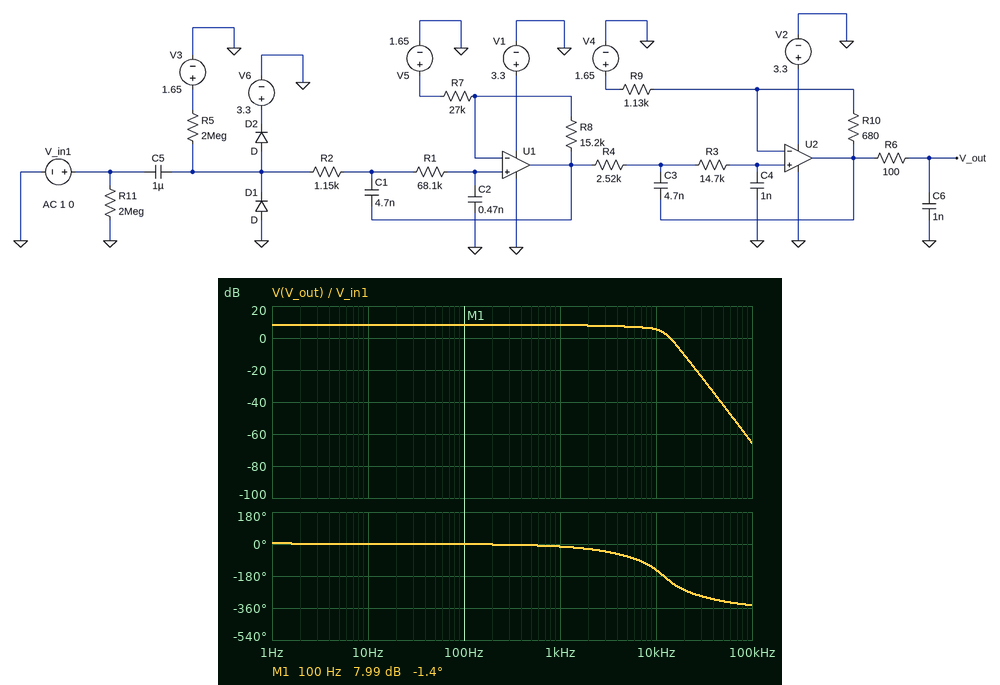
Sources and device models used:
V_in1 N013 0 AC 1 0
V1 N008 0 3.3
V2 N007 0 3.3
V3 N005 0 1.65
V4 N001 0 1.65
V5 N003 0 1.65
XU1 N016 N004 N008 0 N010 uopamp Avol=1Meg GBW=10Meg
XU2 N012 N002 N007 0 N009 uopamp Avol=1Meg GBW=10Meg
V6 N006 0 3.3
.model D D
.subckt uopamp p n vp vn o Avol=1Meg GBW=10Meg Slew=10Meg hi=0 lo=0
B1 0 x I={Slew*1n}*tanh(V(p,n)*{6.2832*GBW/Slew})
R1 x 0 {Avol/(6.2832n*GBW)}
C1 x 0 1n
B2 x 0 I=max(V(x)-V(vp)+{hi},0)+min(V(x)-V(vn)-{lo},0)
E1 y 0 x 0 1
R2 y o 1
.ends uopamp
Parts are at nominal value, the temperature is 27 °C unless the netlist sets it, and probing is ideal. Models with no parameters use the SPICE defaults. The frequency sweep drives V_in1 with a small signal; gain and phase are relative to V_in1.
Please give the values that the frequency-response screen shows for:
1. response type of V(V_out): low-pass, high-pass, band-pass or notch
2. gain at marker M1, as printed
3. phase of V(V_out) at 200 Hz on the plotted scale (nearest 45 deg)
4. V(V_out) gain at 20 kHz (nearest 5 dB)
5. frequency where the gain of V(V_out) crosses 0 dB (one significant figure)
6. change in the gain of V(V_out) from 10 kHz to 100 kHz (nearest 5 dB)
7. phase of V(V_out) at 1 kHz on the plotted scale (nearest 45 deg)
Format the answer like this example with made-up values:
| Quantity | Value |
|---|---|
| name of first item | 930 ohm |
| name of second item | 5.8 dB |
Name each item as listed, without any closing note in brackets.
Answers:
| Quantity | Value |
|---|---|
| response type of V(V_out): low-pass, high-pass, band-pass or notch | low-pass |
| gain at marker M1, as printed | 7.99 dB |
| phase of V(V_out) at 200 Hz on the plotted scale | 0 deg |
| V(V_out) gain at 20 kHz | -10 dB |
| frequency where the gain of V(V_out) crosses 0 dB | 10 kHz |
| change in the gain of V(V_out) from 10 kHz to 100 kHz | -70 dB |
| phase of V(V_out) at 1 kHz on the plotted scale | 0 deg |
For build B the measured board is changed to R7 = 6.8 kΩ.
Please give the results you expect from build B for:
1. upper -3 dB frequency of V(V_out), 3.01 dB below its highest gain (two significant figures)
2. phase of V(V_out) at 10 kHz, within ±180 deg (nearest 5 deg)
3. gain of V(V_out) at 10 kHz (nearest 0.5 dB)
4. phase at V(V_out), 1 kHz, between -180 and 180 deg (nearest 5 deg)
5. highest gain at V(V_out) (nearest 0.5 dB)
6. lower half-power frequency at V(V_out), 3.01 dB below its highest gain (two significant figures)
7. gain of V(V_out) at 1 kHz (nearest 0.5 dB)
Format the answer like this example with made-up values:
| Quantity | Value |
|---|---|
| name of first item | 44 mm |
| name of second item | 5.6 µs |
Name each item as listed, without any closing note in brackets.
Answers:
| Quantity | Value |
|---|---|
| upper -3 dB frequency of V(V_out), 3.01 dB below its highest gain | 12 kHz |
| phase of V(V_out) at 10 kHz, within ±180 deg | -140 deg |
| gain of V(V_out) at 10 kHz | 15.0 dB |
| phase at V(V_out), 1 kHz, between -180 and 180 deg | -10 deg |
| highest gain at V(V_out) | 15.5 dB |
| lower half-power frequency at V(V_out), 3.01 dB below its highest gain | 100 mHz |
| gain of V(V_out) at 1 kHz | 14.5 dB |
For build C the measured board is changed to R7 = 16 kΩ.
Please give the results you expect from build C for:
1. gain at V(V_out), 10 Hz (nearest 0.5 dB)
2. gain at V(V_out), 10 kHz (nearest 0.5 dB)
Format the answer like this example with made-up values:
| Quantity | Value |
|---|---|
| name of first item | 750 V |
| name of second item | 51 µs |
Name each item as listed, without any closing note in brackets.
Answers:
| Quantity | Value |
|---|---|
| gain at V(V_out), 10 Hz | 10.0 dB |
| gain at V(V_out), 10 kHz | 8.0 dB |
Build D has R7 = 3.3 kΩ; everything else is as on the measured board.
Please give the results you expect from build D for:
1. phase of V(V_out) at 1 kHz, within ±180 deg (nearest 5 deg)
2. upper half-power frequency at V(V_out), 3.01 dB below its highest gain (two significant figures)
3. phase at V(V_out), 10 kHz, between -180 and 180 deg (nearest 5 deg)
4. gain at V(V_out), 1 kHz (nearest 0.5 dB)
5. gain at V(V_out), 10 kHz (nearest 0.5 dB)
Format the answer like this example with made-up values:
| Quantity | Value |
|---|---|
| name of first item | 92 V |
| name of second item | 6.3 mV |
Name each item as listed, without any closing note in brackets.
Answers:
| Quantity | Value |
|---|---|
| phase of V(V_out) at 1 kHz, within ±180 deg | -5 deg |
| upper half-power frequency at V(V_out), 3.01 dB below its highest gain | 13 kHz |
| phase at V(V_out), 10 kHz, between -180 and 180 deg | -125 deg |
| gain at V(V_out), 1 kHz | 19.5 dB |
| gain at V(V_out), 10 kHz | 27.0 dB |
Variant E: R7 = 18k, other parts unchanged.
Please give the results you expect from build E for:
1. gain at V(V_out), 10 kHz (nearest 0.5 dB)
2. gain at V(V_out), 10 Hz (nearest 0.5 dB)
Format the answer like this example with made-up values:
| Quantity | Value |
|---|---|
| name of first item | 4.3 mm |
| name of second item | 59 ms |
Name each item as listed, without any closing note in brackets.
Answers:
| Quantity | Value |
|---|---|
| gain at V(V_out), 10 kHz | 7.5 dB |
| gain at V(V_out), 10 Hz | 9.5 dB |
